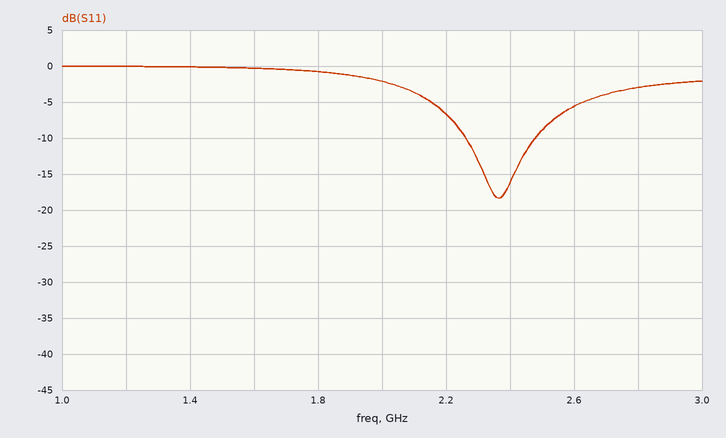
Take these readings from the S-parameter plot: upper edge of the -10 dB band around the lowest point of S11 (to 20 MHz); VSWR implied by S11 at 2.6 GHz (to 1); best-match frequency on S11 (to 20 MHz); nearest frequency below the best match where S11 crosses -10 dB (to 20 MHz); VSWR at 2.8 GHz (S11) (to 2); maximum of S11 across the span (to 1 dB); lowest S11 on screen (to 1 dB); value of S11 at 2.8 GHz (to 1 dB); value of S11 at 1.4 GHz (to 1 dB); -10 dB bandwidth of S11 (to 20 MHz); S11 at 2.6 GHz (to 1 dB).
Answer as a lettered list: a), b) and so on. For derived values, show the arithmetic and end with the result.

a) 2.48 GHz
b) |Γ| = 10^(-6/20) = 0.5012; VSWR = (1 + 0.5012)/(1 − 0.5012) ≈ 3
c) 2.36 GHz
d) 2.26 GHz
e) |Γ| = 10^(-3/20) = 0.7079; VSWR = (1 + 0.7079)/(1 − 0.7079) ≈ 6
f) 0 dB
g) -18 dB
h) -3 dB
i) 0 dB
j) 2.48 GHz − 2.26 GHz = 220 MHz
k) -6 dB
